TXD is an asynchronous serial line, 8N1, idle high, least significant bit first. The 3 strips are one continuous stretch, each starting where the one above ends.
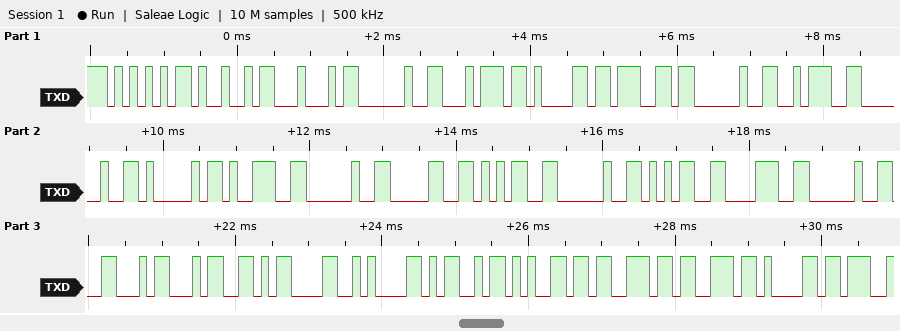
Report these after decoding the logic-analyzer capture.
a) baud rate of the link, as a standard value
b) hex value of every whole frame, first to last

9600 baud
0x55 0x49 0x44 0x20 0x74 0x61 0x67 0x20 0x3A 0x20 0x41 0x39 0x20 0x30 0x35 0x20 0x35 0x38 0x20 0x46 0x34 0x0D 0x0A 0x4D 0x65 0x73 0x73 0x61
